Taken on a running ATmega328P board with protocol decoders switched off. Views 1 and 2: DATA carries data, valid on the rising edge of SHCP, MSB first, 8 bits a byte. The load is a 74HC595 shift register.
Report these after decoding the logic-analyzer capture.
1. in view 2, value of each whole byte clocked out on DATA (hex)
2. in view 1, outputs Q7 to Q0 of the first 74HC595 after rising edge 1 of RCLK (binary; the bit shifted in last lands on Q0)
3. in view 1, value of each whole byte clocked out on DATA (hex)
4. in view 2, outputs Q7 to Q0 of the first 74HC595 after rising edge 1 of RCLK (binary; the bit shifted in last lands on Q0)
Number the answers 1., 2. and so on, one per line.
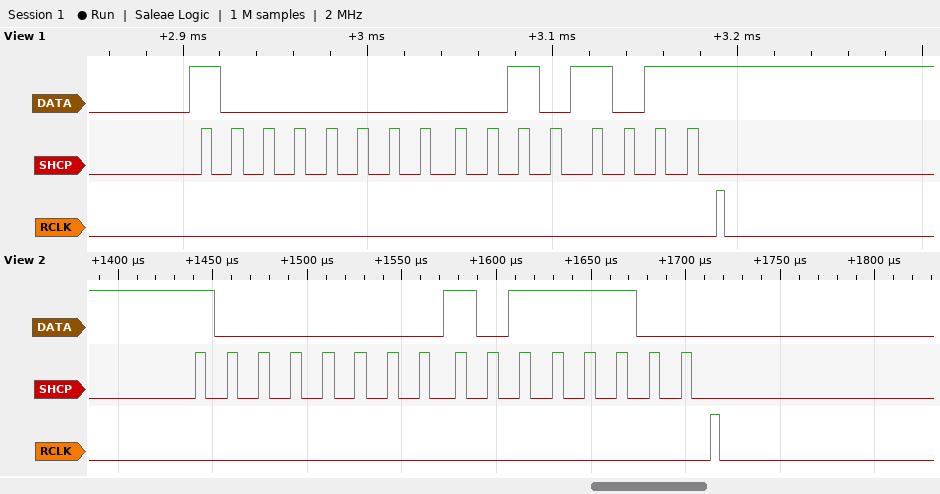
1. 0x80 0xBC
2. 00101011
3. 80 2B
4. 10111100
